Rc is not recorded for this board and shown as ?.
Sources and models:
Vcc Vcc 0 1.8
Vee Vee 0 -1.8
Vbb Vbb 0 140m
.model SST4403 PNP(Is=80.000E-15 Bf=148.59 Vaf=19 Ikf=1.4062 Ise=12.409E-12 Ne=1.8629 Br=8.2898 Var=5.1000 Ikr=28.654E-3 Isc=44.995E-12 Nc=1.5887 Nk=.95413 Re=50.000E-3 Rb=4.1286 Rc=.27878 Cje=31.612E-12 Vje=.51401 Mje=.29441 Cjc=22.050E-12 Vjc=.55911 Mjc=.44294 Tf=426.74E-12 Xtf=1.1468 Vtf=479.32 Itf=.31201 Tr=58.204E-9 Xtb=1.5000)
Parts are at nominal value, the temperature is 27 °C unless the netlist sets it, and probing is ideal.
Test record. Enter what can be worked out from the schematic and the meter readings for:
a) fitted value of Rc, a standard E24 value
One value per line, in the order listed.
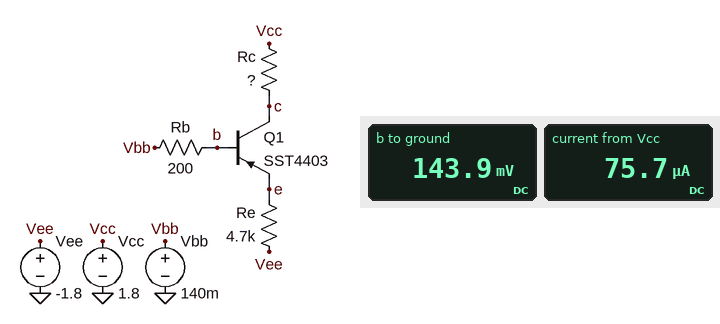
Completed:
15 kΩ
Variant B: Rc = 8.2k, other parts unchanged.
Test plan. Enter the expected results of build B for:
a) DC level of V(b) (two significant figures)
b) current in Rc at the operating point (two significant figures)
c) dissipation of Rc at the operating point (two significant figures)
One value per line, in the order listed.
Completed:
150 mV
140 µA
150 µW
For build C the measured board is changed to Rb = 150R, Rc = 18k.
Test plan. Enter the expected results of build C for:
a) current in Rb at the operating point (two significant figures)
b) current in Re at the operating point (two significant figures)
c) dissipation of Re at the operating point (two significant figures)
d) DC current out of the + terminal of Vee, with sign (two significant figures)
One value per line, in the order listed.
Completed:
17 µA
47 µA
10 µW
-47 µA
